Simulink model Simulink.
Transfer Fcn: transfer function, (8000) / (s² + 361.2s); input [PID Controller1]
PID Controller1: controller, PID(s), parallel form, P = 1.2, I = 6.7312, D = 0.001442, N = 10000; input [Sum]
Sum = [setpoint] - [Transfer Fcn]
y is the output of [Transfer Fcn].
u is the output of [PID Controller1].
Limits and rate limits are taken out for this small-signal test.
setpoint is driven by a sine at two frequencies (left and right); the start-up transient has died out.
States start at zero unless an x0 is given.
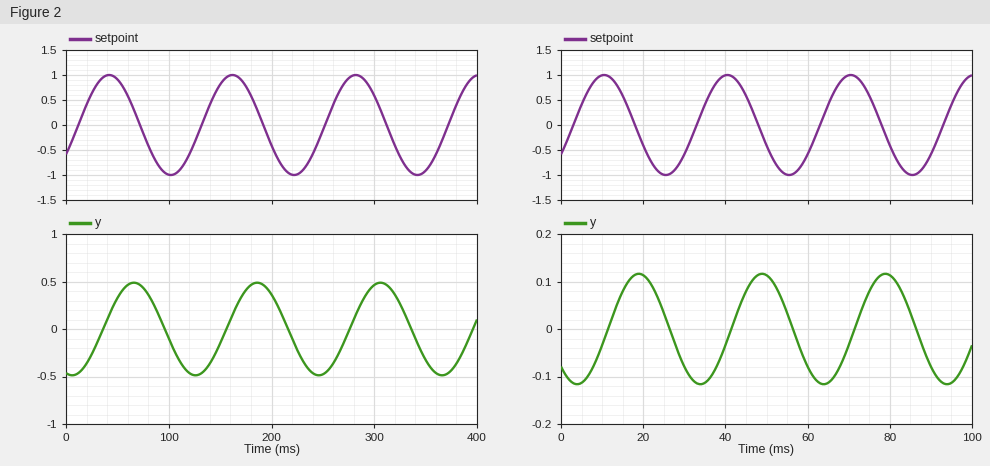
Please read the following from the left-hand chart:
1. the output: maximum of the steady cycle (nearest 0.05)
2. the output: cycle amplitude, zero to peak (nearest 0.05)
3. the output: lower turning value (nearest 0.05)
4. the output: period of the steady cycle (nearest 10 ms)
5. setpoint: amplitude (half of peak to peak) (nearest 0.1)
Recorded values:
0.50
0.50
-0.50
120 ms
1.0
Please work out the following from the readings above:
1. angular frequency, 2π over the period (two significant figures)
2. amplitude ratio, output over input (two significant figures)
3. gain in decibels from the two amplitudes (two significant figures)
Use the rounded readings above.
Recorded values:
0.052 rad/ms
0.50
-6.0 dB
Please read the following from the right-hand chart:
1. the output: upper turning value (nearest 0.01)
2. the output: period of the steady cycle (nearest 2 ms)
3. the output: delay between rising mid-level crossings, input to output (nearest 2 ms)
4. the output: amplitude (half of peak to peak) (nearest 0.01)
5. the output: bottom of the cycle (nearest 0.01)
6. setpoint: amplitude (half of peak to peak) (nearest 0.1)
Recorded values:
0.12
30 ms
8 ms
0.12
-0.12
1.0
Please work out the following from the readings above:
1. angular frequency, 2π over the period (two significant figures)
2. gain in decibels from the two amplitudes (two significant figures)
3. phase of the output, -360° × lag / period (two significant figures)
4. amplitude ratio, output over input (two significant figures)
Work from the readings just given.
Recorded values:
0.21 rad/ms
-18 dB
-96°
0.12
